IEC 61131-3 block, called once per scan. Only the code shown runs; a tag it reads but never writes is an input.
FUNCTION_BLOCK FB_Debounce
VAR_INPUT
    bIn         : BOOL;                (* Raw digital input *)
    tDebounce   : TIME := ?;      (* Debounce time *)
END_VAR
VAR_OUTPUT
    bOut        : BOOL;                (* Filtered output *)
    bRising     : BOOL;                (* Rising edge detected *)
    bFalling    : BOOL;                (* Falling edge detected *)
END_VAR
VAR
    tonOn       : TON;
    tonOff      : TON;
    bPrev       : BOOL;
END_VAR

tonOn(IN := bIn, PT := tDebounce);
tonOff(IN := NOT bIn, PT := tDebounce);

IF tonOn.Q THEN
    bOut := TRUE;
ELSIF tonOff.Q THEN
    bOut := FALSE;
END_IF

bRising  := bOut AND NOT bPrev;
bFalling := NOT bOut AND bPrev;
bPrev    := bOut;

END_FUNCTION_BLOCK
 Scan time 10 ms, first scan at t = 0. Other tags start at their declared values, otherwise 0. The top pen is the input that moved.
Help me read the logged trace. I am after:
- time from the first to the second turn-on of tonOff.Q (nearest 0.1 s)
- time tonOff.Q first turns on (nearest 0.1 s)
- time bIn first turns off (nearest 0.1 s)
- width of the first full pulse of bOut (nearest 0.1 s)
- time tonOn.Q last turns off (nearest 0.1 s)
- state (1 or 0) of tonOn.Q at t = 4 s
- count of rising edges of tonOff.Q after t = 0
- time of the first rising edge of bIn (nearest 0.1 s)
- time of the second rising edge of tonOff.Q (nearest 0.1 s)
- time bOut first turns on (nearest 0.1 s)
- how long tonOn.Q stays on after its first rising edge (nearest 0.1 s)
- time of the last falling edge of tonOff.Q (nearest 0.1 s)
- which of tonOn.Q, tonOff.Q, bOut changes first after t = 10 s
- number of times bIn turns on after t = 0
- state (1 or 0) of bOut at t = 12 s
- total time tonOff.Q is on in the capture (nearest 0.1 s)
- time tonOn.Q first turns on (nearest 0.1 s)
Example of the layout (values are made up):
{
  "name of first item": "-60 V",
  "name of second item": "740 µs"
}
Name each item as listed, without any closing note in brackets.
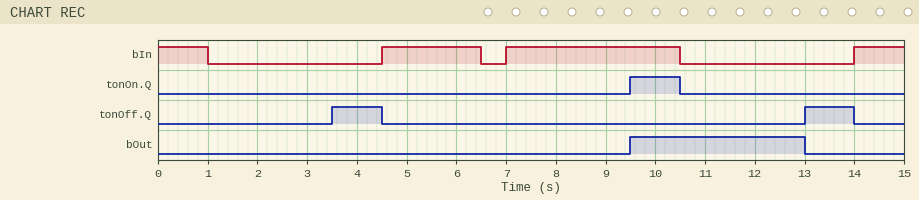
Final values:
{
  "time from the first to the second turn-on of tonOff.Q": "9.5 s",
  "time tonOff.Q first turns on": "3.5 s",
  "time bIn first turns off": "1.0 s",
  "width of the first full pulse of bOut": "3.5 s",
  "time tonOn.Q last turns off": "10.5 s",
  "state (1 or 0) of tonOn.Q at t = 4 s": "0",
  "count of rising edges of tonOff.Q after t = 0": "2",
  "time of the first rising edge of bIn": "4.5 s",
  "time of the second rising edge of tonOff.Q": "13.0 s",
  "time bOut first turns on": "9.5 s",
  "how long tonOn.Q stays on after its first rising edge": "1.0 s",
  "time of the last falling edge of tonOff.Q": "14.0 s",
  "which of tonOn.Q, tonOff.Q, bOut changes first after t = 10 s": "tonOn.Q",
  "number of times bIn turns on after t = 0": "3",
  "state (1 or 0) of bOut at t = 12 s": "1",
  "total time tonOff.Q is on in the capture": "2.0 s",
  "time tonOn.Q first turns on": "9.5 s"
}
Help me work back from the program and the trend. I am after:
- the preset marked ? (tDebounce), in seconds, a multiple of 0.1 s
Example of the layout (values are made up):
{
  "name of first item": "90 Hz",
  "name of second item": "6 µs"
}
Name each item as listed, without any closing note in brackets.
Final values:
{
  "the preset marked ? (tDebounce), in seconds, a multiple of 0.1 s": "2.5 s"
}
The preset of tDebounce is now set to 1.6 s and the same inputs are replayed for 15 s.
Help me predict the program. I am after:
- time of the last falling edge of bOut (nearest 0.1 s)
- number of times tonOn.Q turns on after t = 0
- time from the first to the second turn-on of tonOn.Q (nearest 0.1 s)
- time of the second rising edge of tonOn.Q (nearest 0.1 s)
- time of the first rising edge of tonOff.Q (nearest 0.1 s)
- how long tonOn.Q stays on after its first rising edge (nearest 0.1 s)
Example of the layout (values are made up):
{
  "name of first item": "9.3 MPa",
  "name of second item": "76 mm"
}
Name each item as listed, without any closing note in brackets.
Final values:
{
  "time of the last falling edge of bOut": "12.1 s",
  "number of times tonOn.Q turns on after t = 0": "2",
  "time from the first to the second turn-on of tonOn.Q": "2.5 s",
  "time of the second rising edge of tonOn.Q": "8.6 s",
  "time of the first rising edge of tonOff.Q": "2.6 s",
  "how long tonOn.Q stays on after its first rising edge": "0.4 s"
}
